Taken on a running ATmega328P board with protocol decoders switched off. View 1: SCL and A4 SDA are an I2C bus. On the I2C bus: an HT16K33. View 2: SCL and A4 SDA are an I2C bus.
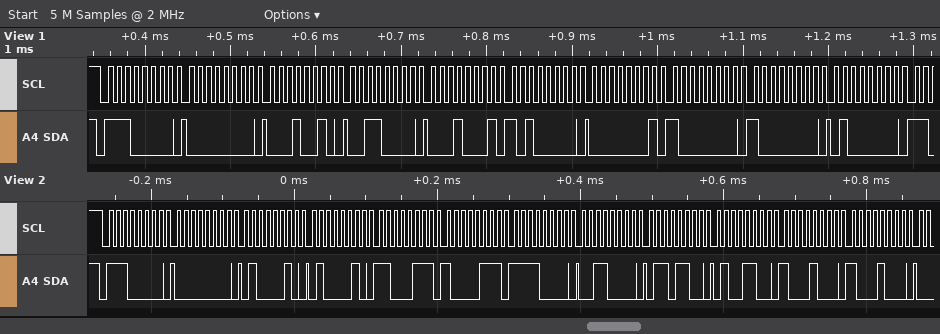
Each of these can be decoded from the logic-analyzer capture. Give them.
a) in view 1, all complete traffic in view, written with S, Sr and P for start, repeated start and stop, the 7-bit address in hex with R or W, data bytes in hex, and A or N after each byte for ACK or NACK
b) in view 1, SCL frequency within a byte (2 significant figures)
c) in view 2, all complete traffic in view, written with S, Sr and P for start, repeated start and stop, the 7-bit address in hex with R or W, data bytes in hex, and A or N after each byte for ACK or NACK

S 70W A 00 A 12 A 30 A 11 A A0 A 01 A 80 A 80 A 40 A
100 kHz
S 70W A 00 A 42 A 42 A C7 A 87 A F0 A 30 A 6C A 4C A 88 A 88 A
